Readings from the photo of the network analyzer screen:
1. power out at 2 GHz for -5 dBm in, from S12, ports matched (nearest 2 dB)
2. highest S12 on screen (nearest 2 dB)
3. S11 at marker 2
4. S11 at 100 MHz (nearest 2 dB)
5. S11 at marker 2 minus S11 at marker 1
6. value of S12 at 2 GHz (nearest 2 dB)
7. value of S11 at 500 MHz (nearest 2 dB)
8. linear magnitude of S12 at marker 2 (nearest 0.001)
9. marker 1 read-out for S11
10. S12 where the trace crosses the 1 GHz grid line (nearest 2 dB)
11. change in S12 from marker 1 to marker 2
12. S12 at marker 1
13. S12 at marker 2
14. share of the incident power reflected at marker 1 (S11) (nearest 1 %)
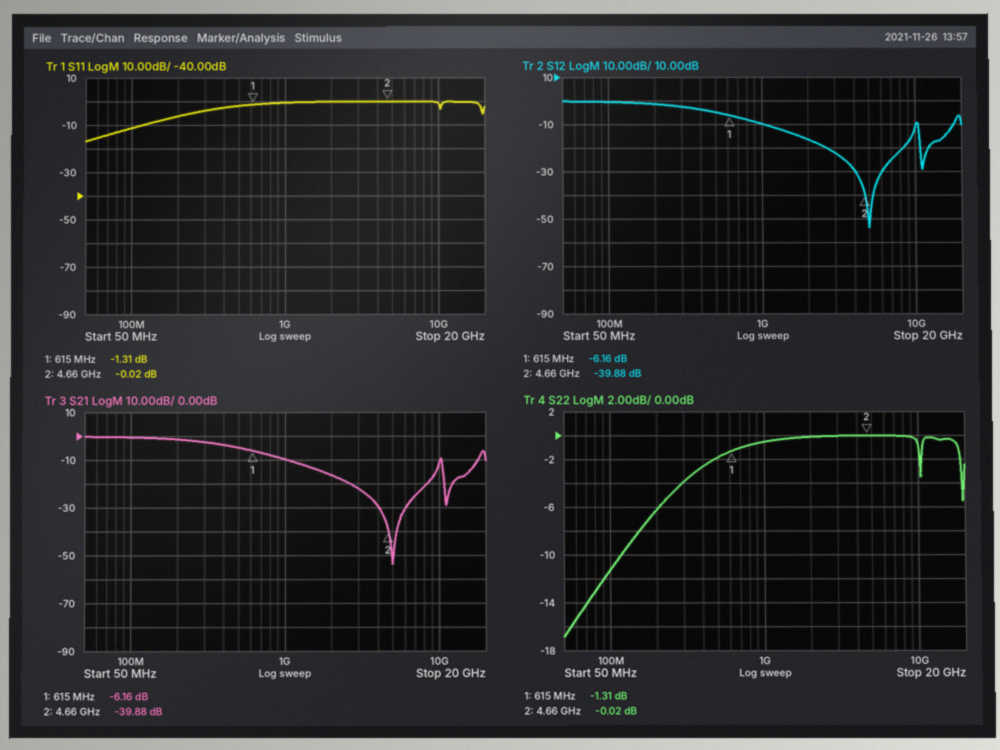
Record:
-22 dBm
0 dB
-0.02 dB
-12 dB
1.29 dB
-16 dB
-2 dB
0.010
-1.31 dB
-10 dB
-33.72 dB
-6.16 dB
-39.88 dB
74 %
